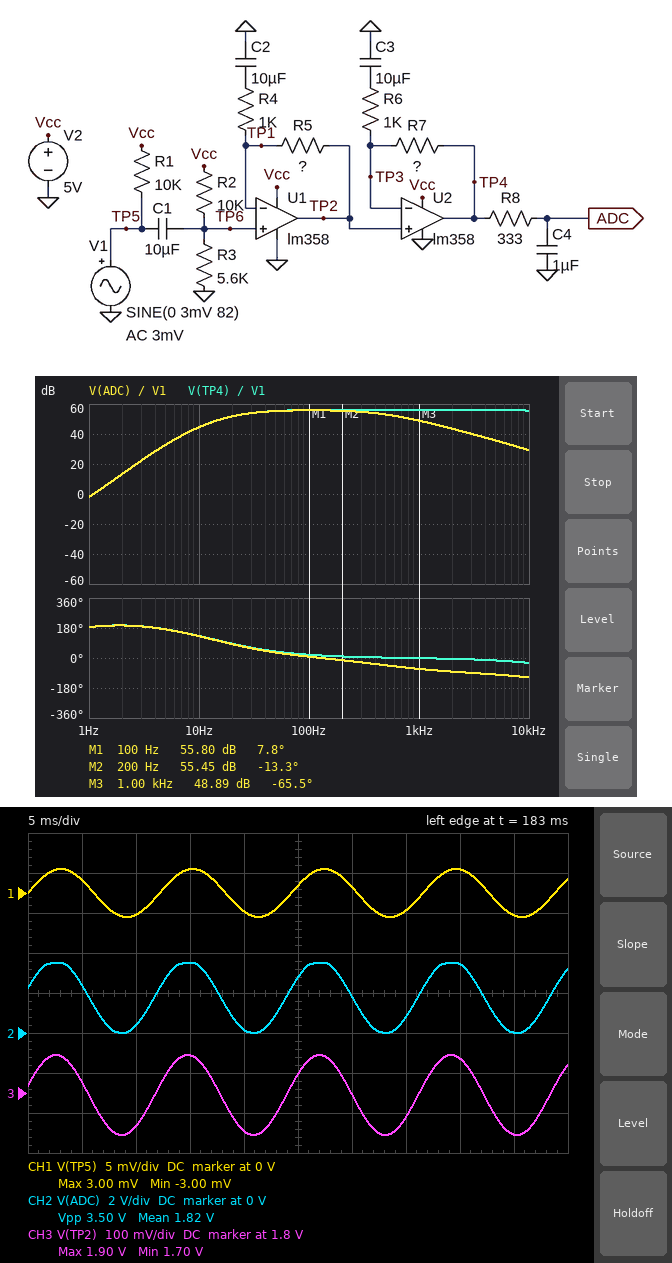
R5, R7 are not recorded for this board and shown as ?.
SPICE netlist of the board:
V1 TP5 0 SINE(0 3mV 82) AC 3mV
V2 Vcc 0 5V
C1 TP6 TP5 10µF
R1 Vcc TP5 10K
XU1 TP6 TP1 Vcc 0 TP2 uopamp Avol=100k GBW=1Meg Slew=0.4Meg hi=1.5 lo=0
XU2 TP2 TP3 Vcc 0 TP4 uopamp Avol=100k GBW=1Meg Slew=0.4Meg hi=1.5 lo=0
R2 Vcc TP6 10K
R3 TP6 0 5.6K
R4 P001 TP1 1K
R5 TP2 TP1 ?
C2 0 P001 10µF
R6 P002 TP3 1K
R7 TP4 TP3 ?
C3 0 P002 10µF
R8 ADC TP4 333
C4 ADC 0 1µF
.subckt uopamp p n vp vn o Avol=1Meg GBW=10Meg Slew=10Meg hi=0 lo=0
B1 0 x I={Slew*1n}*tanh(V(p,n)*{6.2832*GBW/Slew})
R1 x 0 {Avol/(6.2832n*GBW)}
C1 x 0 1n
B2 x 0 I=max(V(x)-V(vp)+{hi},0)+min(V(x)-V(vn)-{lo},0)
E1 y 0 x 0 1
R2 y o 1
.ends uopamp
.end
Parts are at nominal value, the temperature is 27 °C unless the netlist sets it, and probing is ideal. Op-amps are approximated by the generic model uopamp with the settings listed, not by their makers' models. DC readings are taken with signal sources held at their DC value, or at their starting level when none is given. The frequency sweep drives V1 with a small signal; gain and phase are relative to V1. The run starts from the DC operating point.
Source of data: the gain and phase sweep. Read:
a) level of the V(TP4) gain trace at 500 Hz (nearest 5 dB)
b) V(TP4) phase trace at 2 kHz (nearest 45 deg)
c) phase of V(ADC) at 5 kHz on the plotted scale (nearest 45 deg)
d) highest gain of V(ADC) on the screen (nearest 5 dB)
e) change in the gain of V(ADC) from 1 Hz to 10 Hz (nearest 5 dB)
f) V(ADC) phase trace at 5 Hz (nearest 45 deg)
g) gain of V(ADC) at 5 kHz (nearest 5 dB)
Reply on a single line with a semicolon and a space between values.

55 dB; 0 deg; -90 deg; 55 dB; 45 dB; 180 deg; 35 dB
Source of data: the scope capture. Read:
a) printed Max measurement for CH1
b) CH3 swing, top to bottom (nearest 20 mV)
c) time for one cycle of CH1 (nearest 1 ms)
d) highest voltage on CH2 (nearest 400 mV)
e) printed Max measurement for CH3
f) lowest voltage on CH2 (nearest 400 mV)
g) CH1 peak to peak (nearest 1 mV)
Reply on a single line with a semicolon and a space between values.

3.00 mV; 200 mV; 12 ms; 3.6 V; 1.90 V; 0 V; 6 mV
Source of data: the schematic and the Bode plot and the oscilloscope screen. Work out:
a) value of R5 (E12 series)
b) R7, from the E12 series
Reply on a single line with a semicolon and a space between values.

33 kΩ; 18 kΩ
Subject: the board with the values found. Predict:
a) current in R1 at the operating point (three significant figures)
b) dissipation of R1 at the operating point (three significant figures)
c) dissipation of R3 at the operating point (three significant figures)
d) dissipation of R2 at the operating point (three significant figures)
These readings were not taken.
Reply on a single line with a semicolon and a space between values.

500 µA; 2.50 mW; 575 µW; 1.03 mW
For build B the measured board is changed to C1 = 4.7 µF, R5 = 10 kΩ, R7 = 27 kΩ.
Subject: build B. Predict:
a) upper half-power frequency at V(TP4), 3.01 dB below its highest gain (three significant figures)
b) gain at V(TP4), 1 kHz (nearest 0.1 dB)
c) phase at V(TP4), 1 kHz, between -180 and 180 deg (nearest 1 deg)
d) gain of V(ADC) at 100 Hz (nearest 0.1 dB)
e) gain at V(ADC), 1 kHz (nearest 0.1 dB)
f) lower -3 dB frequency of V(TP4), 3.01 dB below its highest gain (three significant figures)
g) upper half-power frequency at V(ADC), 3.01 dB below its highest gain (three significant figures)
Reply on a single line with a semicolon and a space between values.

31.6 kHz; 49.8 dB; 0 deg; 49.3 dB; 42.5 dB; 27.3 Hz; 525 Hz
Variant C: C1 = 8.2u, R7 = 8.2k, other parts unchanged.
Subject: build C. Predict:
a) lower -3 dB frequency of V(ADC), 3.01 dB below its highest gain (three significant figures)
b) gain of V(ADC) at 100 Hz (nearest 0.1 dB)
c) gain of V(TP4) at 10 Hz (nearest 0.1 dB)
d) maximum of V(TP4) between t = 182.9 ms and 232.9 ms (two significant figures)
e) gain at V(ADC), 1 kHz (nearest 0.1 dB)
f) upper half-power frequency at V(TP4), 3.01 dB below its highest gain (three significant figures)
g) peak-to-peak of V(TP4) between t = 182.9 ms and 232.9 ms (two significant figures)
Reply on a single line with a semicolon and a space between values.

23.8 Hz; 49.5 dB; 38.0 dB; 2.7 V; 42.6 dB; 27.6 kHz; 1.8 V
